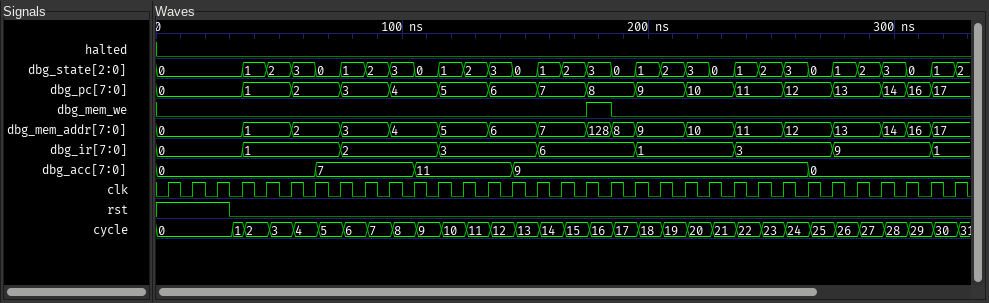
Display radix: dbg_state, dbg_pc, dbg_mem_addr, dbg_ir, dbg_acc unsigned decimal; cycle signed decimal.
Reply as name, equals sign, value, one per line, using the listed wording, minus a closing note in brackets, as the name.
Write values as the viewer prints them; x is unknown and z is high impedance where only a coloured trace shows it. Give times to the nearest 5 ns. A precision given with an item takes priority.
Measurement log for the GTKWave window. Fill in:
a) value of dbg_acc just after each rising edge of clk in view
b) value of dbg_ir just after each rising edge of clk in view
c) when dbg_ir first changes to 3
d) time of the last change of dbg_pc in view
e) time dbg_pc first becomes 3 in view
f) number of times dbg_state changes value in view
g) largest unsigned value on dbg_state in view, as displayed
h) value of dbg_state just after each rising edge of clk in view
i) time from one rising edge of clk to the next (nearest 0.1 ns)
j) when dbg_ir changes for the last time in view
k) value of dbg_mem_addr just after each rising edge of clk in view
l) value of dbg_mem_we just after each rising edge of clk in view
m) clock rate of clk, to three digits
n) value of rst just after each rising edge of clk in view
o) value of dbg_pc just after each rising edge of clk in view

value of dbg_acc just after each rising edge of clk in view = 0, 0, 0, 0, 0, 0, 7, 7, 7, 7, 11, 11, 11, 11, 9, 9, 9, 9, 9, 9, 9, 9, 9, 9, 9, 9, 0, 0, 0, 0, 0, 0, 0
value of dbg_ir just after each rising edge of clk in view = 0, 0, 0, 1, 1, 1, 1, 2, 2, 2, 2, 3, 3, 3, 3, 6, 6, 6, 6, 1, 1, 1, 1, 3, 3, 3, 3, 9, 9, 9, 9, 1, 1
when dbg_ir first changes to 3 = 115 ns
time of the last change of dbg_pc in view = 315 ns
time dbg_pc first becomes 3 in view = 75 ns
number of times dbg_state changes value in view = 30
largest unsigned value on dbg_state in view, as displayed = 3
value of dbg_state just after each rising edge of clk in view = 0, 0, 0, 1, 2, 3, 0, 1, 2, 3, 0, 1, 2, 3, 0, 1, 2, 3, 0, 1, 2, 3, 0, 1, 2, 3, 0, 1, 2, 3, 0, 1, 2
time from one rising edge of clk to the next = 10 ns
when dbg_ir changes for the last time in view = 315 ns
value of dbg_mem_addr just after each rising edge of clk in view = 0, 0, 0, 1, 1, 2, 2, 3, 3, 4, 4, 5, 5, 6, 6, 7, 7, 128, 8, 9, 9, 10, 10, 11, 11, 12, 12, 13, 13, 14, 16, 17, 17
value of dbg_mem_we just after each rising edge of clk in view = 0 0 0 0 0 0 0 0 0 0 0 0 0 0 0 0 0 1 0 0 0 0 0 0 0 0 0 0 0 0 0 0 0
clock rate of clk, to three digits = 100 MHz
value of rst just after each rising edge of clk in view = 1 1 1 0 0 0 0 0 0 0 0 0 0 0 0 0 0 0 0 0 0 0 0 0 0 0 0 0 0 0 0 0 0
value of dbg_pc just after each rising edge of clk in view = 0, 0, 0, 1, 1, 2, 2, 3, 3, 4, 4, 5, 5, 6, 6, 7, 7, 8, 8, 9, 9, 10, 10, 11, 11, 12, 12, 13, 13, 14, 16, 17, 17
